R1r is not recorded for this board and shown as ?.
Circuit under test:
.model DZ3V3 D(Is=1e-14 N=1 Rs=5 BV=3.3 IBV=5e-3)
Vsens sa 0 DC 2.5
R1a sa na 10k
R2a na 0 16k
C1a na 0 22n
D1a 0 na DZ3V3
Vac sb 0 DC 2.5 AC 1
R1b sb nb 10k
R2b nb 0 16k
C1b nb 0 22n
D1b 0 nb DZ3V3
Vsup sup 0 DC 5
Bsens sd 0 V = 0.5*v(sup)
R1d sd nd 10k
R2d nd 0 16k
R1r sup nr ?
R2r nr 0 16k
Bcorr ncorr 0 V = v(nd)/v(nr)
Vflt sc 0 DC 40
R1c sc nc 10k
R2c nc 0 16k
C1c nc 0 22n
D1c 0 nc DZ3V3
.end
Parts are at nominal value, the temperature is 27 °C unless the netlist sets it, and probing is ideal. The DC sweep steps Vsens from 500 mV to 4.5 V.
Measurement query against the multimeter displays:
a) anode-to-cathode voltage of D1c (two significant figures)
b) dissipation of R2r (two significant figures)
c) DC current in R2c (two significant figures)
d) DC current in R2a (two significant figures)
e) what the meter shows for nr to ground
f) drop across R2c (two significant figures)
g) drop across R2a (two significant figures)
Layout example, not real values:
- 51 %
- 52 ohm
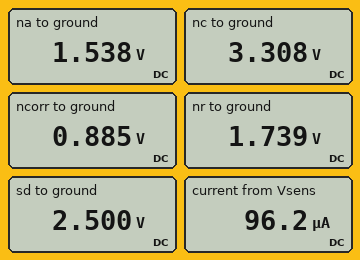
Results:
- -3.3 V
- 190 µW
- 210 µA
- 96 µA
- 1.739 V
- 3.3 V
- 1.5 V
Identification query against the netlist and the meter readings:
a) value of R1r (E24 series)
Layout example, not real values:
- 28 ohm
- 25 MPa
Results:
- 30 kΩ
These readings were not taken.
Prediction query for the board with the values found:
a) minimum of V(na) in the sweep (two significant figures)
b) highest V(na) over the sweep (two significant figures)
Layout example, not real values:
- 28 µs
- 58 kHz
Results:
- 310 mV
- 2.8 V
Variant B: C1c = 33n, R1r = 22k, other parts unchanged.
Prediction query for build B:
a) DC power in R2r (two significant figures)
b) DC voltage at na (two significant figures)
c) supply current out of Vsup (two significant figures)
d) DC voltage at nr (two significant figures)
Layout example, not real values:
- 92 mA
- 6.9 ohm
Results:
- 280 µW
- 1.5 V
- 130 µA
- 2.1 V
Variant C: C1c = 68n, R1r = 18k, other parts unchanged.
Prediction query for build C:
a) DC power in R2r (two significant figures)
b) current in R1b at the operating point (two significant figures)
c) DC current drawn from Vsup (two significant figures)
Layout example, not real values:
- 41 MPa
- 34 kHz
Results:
- 350 µW
- 96 µA
- 150 µA
